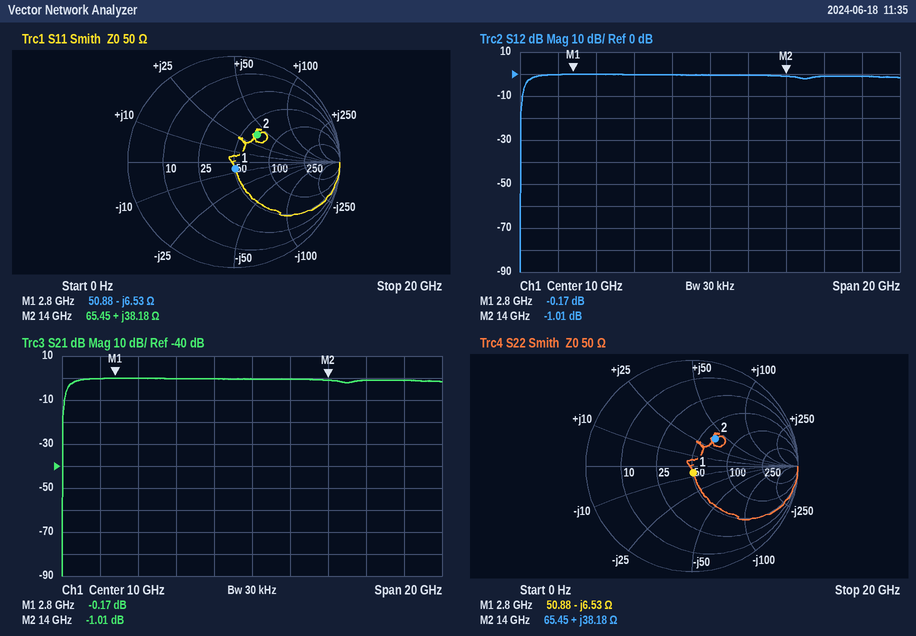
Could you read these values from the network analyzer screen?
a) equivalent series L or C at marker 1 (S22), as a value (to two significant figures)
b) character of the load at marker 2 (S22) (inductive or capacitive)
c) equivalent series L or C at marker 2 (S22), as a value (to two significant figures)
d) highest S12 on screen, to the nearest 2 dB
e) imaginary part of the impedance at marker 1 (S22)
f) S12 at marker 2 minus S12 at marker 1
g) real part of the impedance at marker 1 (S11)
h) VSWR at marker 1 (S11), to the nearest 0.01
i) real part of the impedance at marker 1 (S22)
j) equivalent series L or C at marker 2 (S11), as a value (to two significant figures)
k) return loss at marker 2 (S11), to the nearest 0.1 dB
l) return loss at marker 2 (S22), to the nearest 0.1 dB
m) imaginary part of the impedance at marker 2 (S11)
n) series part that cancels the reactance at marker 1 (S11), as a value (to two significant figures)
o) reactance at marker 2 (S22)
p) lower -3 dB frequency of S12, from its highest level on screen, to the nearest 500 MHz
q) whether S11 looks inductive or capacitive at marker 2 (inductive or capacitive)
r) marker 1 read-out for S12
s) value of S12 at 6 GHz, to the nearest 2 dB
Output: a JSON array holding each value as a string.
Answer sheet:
["8.7 pF", "inductive", "430 pH", "0 dB", "-6.53 Ω", "-0.84 dB", "50.88 Ω", "1.14", "50.88 Ω", "430 pH", "9.4 dB", "9.4 dB", "+38.18 Ω", "370 pH", "+38.18 Ω", "500 MHz", "inductive", "-0.17 dB", "0 dB"]
